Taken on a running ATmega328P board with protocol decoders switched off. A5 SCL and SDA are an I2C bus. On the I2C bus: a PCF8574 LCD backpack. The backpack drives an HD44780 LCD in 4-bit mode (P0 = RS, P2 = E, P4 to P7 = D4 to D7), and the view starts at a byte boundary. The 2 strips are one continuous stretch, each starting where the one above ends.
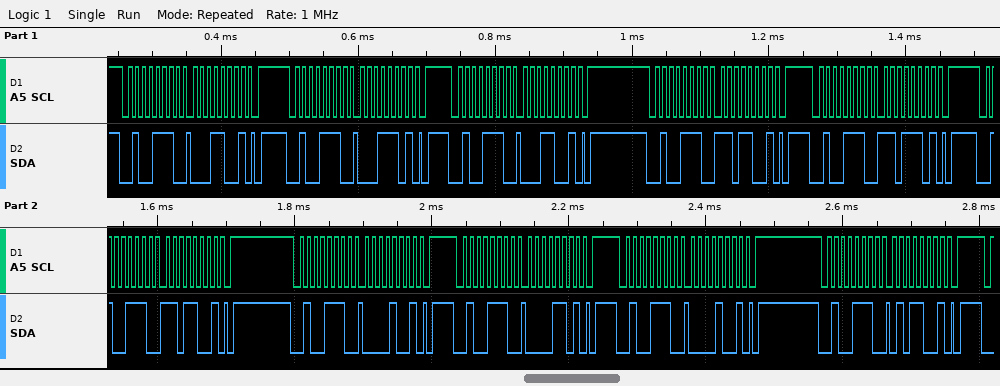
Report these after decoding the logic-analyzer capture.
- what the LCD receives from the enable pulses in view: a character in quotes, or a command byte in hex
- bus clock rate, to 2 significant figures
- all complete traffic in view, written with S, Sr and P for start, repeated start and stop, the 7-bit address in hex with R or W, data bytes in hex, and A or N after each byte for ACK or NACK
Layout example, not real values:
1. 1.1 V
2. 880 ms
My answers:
1. data 0x1D
2. 100 kHz
3. S 27W A 19 A P S 27W A 1D A P S 27W A 19 A P S 27W A D9 A P S 27W A DD A P S 27W A D9 A P S 27W A 09 A P S 27W A 0D A P S 27W A 09 A P S 27W A 59 A P
